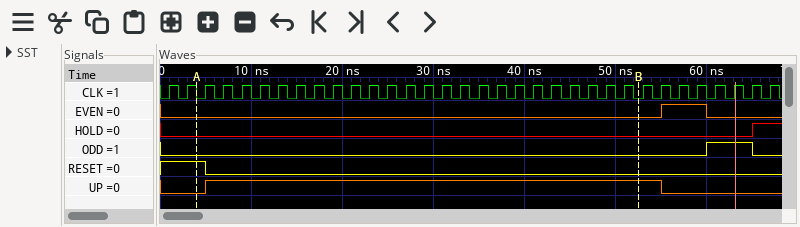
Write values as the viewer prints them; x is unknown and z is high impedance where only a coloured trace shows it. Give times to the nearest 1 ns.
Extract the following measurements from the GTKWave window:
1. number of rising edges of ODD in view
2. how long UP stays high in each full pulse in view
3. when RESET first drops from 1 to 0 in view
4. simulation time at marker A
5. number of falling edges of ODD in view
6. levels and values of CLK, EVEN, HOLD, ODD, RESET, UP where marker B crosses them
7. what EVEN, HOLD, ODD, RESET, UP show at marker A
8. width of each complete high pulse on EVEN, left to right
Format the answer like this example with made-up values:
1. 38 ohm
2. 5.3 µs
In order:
1. 1
2. 50 ns
3. 5 ns
4. 4 ns
5. 1
6. CLK=0, EVEN=0, HOLD=0, ODD=0, RESET=0, UP=1
7. EVEN=0, HOLD=0, ODD=0, RESET=1, UP=0
8. 5 ns
